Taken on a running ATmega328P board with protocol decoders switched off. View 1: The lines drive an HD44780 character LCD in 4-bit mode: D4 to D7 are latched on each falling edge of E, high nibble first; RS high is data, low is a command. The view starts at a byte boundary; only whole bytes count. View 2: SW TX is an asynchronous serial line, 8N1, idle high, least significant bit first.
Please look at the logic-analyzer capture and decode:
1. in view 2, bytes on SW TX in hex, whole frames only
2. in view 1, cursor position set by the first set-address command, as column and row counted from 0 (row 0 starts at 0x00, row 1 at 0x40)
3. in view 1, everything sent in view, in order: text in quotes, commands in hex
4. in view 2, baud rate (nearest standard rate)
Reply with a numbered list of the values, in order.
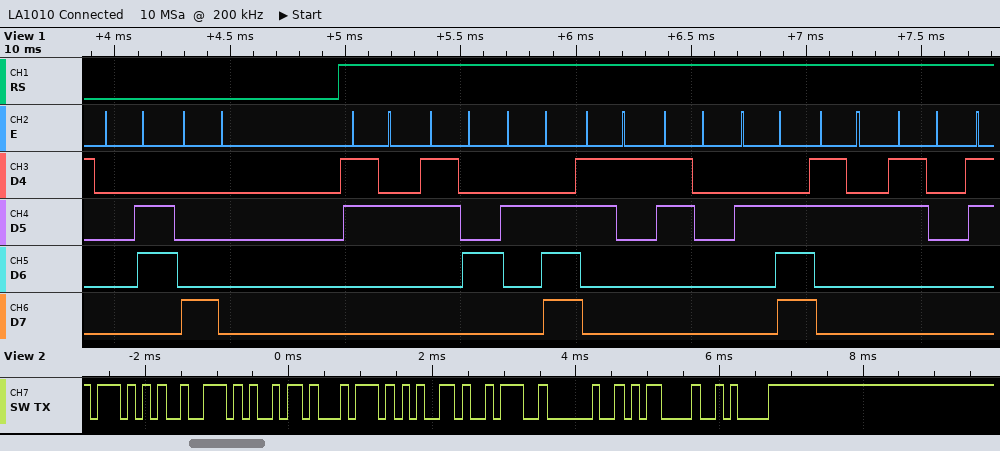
1. 57 72 69 74 65 3A 20 0D 0A
2. column 0, row 0
3. 0x06 0x80 "24.10.20"
4. 9600 baud
